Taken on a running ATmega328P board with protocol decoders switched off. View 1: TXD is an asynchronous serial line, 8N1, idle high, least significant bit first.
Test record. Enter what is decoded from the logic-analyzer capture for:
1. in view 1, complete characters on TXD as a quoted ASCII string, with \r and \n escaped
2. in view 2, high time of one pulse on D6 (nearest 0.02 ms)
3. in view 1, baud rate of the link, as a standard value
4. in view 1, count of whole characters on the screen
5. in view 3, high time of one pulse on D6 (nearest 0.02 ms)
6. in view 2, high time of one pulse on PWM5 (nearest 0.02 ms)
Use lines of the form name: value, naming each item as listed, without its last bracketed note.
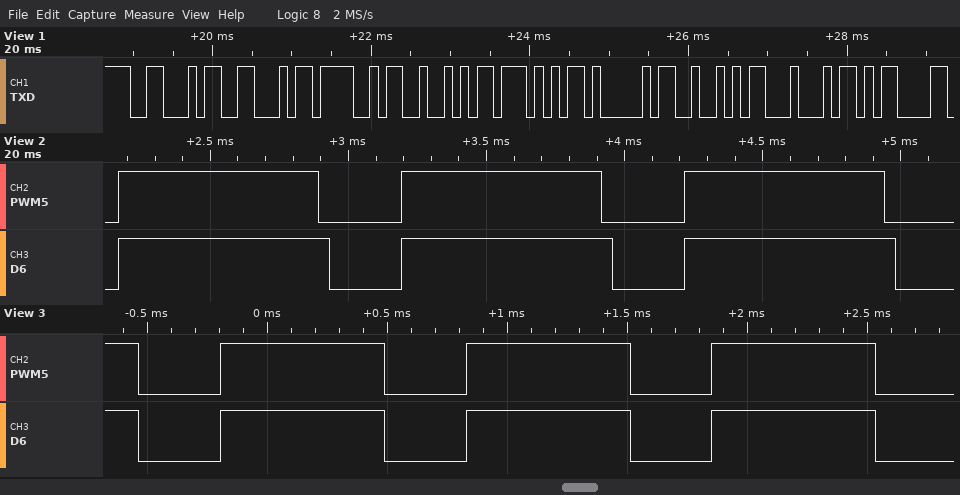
in view 1, complete characters on TXD as a quoted ASCII string, with \r and \n escaped: "FFORWARD\r"
in view 2, high time of one pulse on D6: 0.76 ms
in view 1, baud rate of the link, as a standard value: 9600 baud
in view 1, count of whole characters on the screen: 9
in view 3, high time of one pulse on D6: 0.68 ms
in view 2, high time of one pulse on PWM5: 0.72 ms
